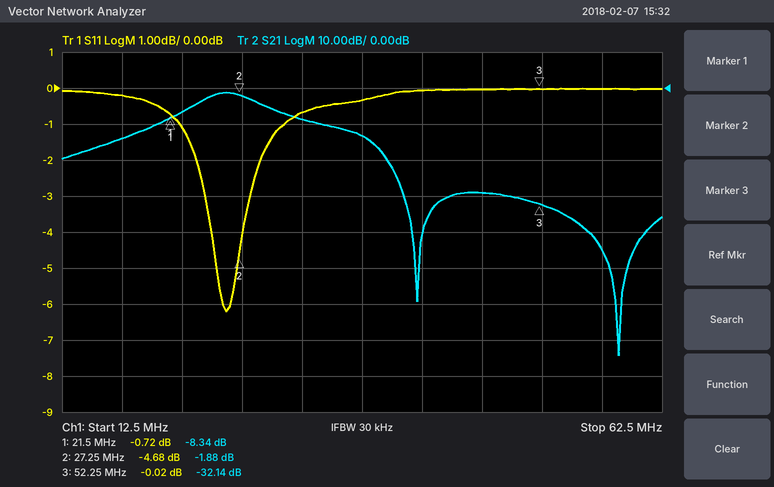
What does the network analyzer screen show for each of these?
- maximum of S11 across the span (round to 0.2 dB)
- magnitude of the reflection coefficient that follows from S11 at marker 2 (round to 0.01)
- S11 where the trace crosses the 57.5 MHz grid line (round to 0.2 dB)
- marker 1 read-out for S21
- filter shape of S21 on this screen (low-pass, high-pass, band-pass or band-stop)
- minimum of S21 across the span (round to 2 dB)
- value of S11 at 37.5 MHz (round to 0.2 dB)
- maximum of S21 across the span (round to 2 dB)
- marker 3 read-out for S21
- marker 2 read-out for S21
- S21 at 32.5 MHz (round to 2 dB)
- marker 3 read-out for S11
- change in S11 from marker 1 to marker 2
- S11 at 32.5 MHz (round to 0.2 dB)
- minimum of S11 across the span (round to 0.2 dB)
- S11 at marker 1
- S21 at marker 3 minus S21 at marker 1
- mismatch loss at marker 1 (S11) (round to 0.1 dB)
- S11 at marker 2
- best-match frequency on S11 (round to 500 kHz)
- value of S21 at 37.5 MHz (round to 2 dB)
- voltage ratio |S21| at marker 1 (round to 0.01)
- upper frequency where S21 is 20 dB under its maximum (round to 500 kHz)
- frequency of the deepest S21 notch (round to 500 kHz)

0.0 dB
0.58
0.0 dB
-8.34 dB
band-pass
-74 dB
-0.4 dB
-2 dB
-32.14 dB
-1.88 dB
-8 dB
-0.02 dB
-3.96 dB
-0.6 dB
-6.2 dB
-0.72 dB
-23.80 dB
8.2 dB
-4.68 dB
26.0 MHz
-14 dB
0.38
40.0 MHz
59.0 MHz
